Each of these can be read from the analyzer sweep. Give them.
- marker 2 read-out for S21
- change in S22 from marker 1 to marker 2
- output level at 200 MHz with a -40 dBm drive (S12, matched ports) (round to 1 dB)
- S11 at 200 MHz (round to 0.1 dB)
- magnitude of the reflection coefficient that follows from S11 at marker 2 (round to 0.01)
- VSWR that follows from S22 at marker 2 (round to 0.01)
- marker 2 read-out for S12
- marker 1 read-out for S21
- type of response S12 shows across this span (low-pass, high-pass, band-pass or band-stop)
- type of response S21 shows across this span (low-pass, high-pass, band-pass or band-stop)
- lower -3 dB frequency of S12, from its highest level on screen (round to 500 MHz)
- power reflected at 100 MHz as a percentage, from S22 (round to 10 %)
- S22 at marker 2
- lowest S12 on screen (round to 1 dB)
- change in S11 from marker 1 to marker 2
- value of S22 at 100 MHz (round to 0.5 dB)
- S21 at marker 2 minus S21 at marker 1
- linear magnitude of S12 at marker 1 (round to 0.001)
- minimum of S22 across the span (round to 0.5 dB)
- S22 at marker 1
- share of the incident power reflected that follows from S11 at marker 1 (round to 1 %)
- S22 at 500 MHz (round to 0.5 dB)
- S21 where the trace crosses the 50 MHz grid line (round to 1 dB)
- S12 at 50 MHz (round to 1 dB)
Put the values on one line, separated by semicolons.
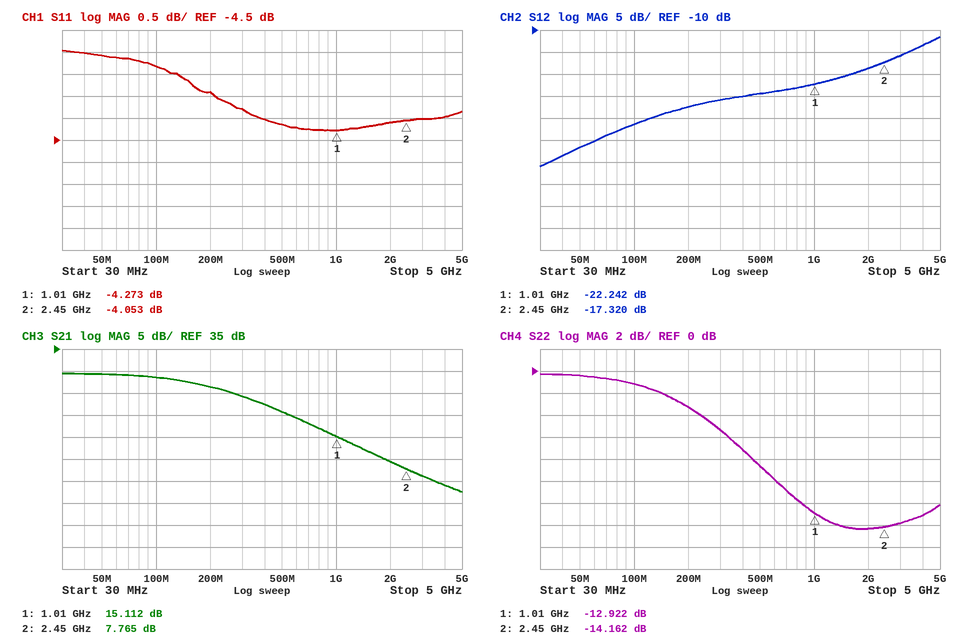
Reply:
7.765 dB; -1.240 dB; -67 dBm; -3.4 dB; 0.63; 1.49; -17.320 dB; 15.112 dB; high-pass; low-pass; 3.5 GHz; 80 %; -14.162 dB; -41 dB; 0.220 dB; -1.0 dB; -7.347 dB; 0.077; -14.5 dB; -12.922 dB; 37 %; -8.5 dB; 29 dB; -37 dB
